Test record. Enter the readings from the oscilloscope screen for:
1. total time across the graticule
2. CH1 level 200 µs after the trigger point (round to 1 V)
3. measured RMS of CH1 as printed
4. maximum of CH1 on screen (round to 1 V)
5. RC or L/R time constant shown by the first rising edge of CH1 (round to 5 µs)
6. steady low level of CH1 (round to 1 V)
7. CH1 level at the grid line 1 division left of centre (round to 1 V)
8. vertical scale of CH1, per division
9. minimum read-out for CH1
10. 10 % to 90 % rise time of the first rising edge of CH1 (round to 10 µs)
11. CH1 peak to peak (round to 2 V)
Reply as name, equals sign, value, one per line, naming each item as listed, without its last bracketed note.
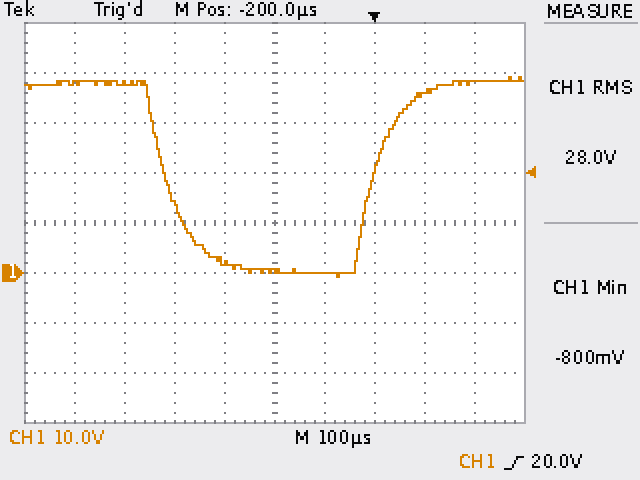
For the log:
total time across the graticule = 1 ms
CH1 level 200 µs after the trigger point = 38 V
measured RMS of CH1 as printed = 28.0 V
maximum of CH1 on screen = 39 V
RC or L/R time constant shown by the first rising edge of CH1 = 50 µs
steady low level of CH1 = 0 V
CH1 level at the grid line 1 division left of centre = 2 V
vertical scale of CH1, per division = 10 V
minimum read-out for CH1 = -800 mV
10 % to 90 % rise time of the first rising edge of CH1 = 110 µs
CH1 peak to peak = 40 V
